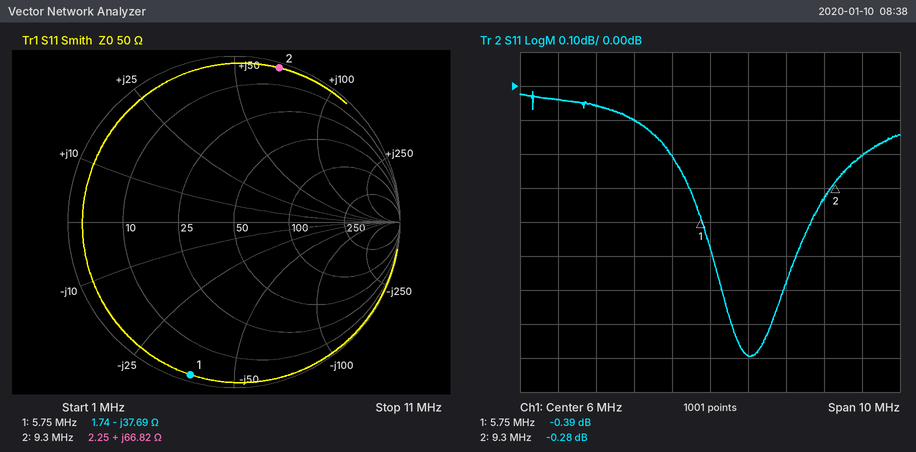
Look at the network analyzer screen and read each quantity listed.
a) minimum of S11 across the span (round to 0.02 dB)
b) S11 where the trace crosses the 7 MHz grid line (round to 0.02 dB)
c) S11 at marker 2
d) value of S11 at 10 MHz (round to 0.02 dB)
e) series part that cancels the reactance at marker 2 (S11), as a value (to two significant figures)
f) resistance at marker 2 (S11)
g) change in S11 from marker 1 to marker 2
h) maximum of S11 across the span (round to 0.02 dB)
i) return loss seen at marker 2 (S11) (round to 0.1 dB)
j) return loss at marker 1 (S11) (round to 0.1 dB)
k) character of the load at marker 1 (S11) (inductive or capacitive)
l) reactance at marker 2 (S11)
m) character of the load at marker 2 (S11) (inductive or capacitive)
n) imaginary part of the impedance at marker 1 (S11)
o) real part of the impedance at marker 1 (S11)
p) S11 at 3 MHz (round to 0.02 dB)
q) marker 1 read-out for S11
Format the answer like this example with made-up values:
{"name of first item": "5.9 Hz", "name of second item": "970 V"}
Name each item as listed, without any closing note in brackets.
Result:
{"minimum of S11 across the span": "-0.80 dB", "S11 where the trace crosses the 7 MHz grid line": "-0.80 dB", "S11 at marker 2": "-0.28 dB", "value of S11 at 10 MHz": "-0.20 dB", "series part that cancels the reactance at marker 2 (S11), as a value": "260 pF", "resistance at marker 2": "2.25 Ω", "change in S11 from marker 1 to marker 2": "0.11 dB", "maximum of S11 across the span": "-0.02 dB", "return loss seen at marker 2 (S11)": "0.3 dB", "return loss at marker 1 (S11)": "0.4 dB", "character of the load at marker 1 (S11)": "capacitive", "reactance at marker 2": "+66.82 Ω", "character of the load at marker 2 (S11)": "inductive", "imaginary part of the impedance at marker 1": "-37.69 Ω", "real part of the impedance at marker 1": "1.74 Ω", "S11 at 3 MHz": "-0.06 dB", "marker 1 read-out for S11": "-0.39 dB"}
